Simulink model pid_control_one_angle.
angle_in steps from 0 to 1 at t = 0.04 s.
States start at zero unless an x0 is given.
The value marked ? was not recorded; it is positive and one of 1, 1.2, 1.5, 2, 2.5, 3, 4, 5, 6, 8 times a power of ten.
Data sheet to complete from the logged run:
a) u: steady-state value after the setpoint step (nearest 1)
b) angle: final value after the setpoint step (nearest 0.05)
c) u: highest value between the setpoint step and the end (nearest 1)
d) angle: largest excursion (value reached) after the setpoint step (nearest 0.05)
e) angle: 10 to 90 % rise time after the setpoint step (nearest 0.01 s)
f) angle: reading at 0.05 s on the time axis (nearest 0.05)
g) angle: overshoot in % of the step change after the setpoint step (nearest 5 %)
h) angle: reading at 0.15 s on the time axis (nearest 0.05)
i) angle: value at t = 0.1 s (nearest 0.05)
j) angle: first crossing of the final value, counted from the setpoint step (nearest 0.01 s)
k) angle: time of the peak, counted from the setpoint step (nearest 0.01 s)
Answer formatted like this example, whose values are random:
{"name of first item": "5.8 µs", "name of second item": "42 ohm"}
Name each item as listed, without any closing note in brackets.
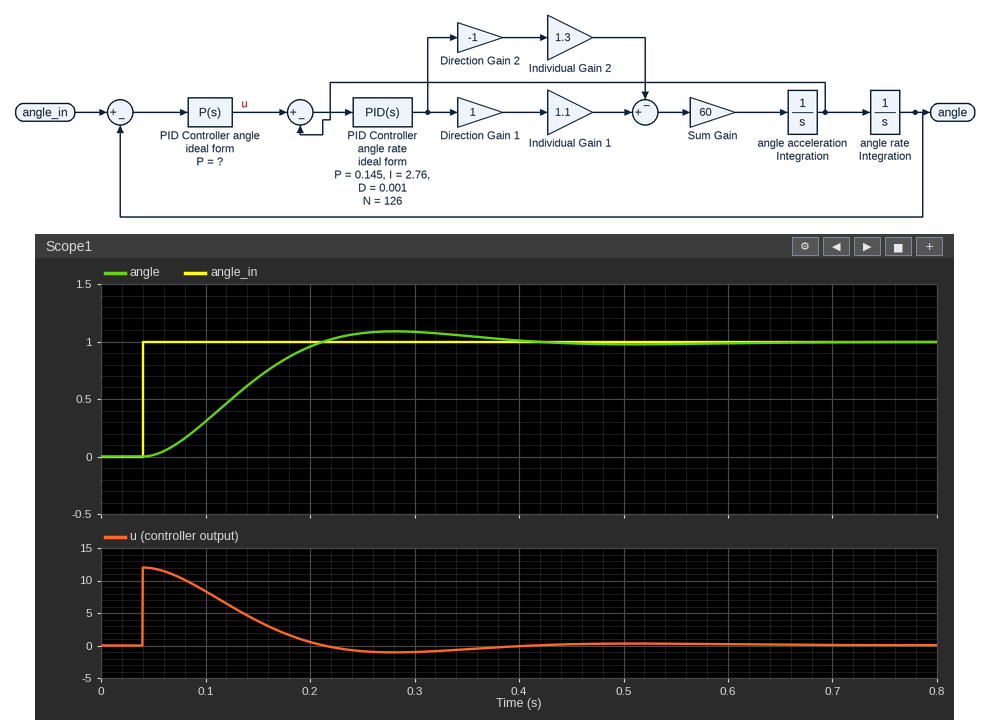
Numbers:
{"u: steady-state value after the setpoint step": "0", "angle: final value after the setpoint step": "1.00", "u: highest value between the setpoint step and the end": "12", "angle: largest excursion (value reached) after the setpoint step": "1.10", "angle: 10 to 90 % rise time after the setpoint step": "0.12 s", "angle: reading at 0.05 s on the time axis": "0.00", "angle: overshoot in % of the step change after the setpoint step": "10 %", "angle: reading at 0.15 s on the time axis": "0.70", "angle: value at t = 0.1 s": "0.30", "angle: first crossing of the final value, counted from the setpoint step": "0.17 s", "angle: time of the peak, counted from the setpoint step": "0.24 s"}
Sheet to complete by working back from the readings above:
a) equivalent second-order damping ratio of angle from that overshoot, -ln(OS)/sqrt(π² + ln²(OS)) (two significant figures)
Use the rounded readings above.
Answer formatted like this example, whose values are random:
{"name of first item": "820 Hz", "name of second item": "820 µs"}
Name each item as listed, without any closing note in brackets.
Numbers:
{"equivalent second-order damping ratio of angle from that overshoot, -ln(OS)/sqrt(π² + ln²(OS))": "0.59"}
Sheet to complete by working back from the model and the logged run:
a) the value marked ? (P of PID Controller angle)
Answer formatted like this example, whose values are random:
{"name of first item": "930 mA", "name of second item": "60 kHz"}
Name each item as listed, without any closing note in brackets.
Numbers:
{"the value marked ?": "12"}
